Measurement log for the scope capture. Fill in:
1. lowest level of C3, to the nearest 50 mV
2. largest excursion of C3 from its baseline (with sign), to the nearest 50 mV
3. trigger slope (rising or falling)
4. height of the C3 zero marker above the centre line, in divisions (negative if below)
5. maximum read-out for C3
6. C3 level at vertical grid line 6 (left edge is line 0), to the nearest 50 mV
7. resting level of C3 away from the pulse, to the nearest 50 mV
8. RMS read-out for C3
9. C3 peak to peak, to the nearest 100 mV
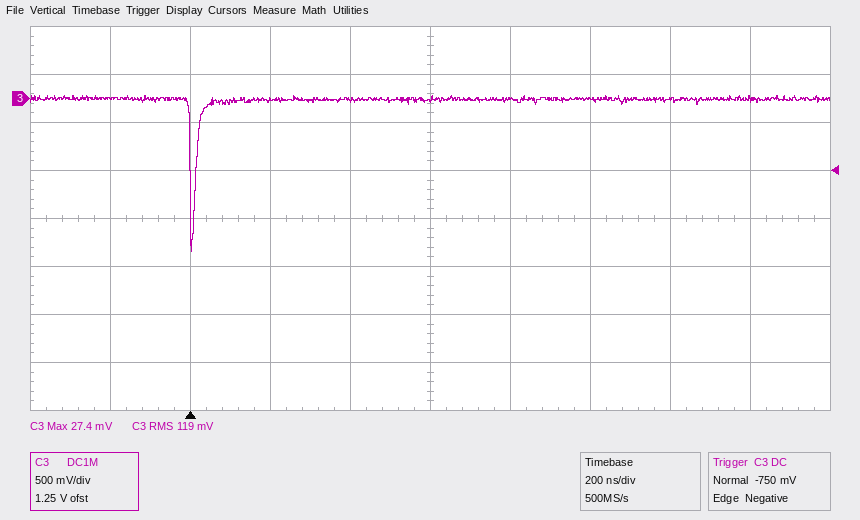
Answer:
-1.60 V
-1.60 V
falling
+2.5 div
27.4 mV
0 mV
0 mV
119 mV
1.60 V
